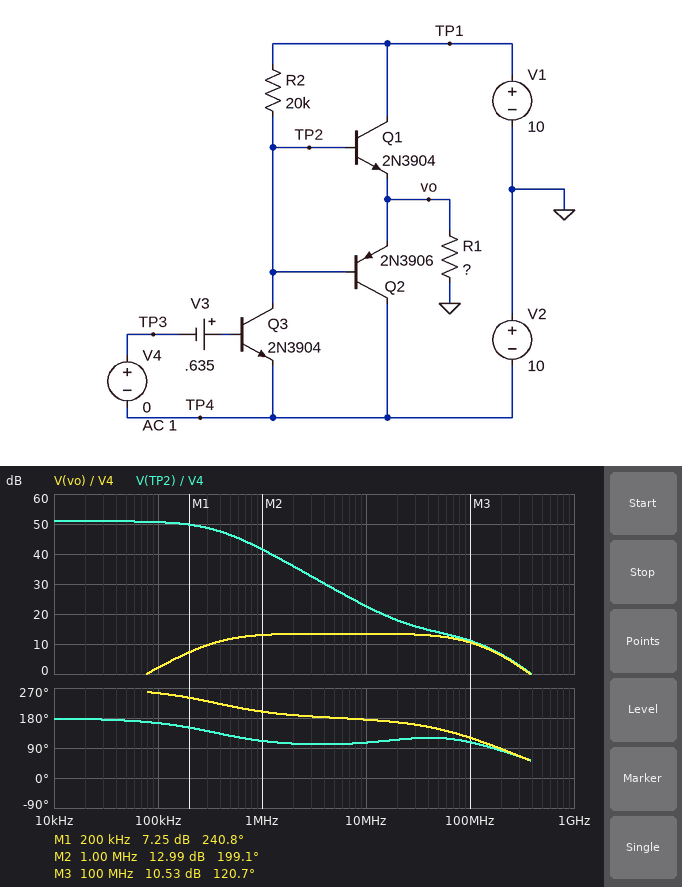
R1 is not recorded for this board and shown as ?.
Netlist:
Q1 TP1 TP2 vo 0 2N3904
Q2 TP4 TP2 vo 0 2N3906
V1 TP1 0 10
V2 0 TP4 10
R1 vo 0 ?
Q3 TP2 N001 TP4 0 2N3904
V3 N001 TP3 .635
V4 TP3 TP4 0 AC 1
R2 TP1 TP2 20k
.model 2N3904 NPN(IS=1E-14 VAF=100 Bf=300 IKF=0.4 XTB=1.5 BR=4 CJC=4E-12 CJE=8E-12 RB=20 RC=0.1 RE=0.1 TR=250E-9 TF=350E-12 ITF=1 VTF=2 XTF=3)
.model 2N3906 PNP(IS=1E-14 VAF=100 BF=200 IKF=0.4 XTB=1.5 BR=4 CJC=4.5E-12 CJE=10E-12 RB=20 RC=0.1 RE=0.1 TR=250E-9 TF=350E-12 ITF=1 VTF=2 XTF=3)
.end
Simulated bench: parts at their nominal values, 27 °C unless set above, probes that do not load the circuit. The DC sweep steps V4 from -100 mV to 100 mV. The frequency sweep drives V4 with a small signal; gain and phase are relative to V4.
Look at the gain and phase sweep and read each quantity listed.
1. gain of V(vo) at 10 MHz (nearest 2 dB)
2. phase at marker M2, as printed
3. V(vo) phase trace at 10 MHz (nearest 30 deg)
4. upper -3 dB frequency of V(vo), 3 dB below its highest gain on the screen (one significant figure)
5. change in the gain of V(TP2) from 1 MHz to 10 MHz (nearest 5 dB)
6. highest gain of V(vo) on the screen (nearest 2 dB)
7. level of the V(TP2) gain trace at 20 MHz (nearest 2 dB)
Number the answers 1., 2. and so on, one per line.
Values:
1. 14 dB
2. 199.1 deg
3. 180 deg
4. 100 MHz
5. -20 dB
6. 14 dB
7. 18 dB
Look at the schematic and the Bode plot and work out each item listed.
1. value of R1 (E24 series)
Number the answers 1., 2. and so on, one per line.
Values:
1. 330 Ω
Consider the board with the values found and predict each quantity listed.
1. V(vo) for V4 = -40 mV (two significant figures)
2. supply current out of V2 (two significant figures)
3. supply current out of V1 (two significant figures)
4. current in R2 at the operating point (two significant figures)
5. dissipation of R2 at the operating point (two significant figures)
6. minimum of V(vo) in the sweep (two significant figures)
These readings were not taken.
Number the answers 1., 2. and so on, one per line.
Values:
1. 5.8 V
2. 500 µA
3. 500 µA
4. 500 µA
5. 5.0 mW
6. -9.2 V
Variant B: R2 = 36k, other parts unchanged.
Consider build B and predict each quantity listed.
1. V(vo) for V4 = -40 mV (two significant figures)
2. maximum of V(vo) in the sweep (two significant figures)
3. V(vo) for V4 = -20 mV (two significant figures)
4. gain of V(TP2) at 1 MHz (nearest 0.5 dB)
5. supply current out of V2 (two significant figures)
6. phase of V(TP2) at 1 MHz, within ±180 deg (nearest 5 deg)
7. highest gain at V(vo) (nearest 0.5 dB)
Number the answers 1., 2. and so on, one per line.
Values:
1. 3.9 V
2. 6.5 V
3. 670 mV
4. 48.5 dB
5. 13 mA
6. 135 deg
7. 51.5 dB
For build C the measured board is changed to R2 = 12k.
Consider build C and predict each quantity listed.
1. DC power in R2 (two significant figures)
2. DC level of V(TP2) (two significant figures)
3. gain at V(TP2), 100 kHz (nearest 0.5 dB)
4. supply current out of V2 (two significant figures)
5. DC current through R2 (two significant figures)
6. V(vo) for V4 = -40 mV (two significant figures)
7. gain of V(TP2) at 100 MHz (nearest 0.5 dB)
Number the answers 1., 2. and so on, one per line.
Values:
1. 3.5 mW
2. 3.5 V
3. 46.0 dB
4. 520 µA
5. 540 µA
6. 7.0 V
7. 13.0 dB
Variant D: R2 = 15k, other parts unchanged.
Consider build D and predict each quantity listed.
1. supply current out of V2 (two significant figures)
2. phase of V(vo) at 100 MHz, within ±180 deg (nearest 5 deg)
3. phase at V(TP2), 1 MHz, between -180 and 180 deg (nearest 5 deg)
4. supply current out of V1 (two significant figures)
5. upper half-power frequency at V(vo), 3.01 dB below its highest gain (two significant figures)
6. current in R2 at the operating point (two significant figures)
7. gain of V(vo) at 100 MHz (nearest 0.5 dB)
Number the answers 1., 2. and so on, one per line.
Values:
1. 510 µA
2. 75 deg
3. 150 deg
4. 4.9 mA
5. 1.8 MHz
6. 520 µA
7. 12.5 dB
